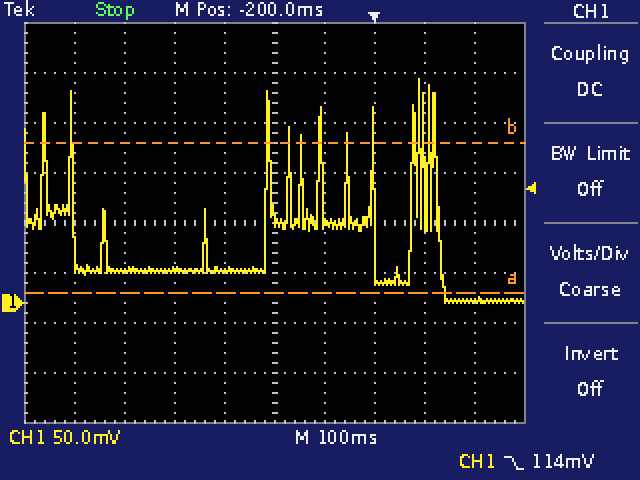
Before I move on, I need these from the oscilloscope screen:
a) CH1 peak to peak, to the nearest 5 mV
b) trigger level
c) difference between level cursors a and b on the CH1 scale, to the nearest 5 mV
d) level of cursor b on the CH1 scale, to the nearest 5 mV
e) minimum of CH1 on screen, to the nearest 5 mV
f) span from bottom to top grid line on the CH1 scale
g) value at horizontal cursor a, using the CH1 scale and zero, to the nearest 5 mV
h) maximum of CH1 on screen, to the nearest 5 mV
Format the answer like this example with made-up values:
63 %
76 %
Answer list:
225 mV
114 mV
150 mV
160 mV
0 mV
400 mV
10 mV
225 mV
